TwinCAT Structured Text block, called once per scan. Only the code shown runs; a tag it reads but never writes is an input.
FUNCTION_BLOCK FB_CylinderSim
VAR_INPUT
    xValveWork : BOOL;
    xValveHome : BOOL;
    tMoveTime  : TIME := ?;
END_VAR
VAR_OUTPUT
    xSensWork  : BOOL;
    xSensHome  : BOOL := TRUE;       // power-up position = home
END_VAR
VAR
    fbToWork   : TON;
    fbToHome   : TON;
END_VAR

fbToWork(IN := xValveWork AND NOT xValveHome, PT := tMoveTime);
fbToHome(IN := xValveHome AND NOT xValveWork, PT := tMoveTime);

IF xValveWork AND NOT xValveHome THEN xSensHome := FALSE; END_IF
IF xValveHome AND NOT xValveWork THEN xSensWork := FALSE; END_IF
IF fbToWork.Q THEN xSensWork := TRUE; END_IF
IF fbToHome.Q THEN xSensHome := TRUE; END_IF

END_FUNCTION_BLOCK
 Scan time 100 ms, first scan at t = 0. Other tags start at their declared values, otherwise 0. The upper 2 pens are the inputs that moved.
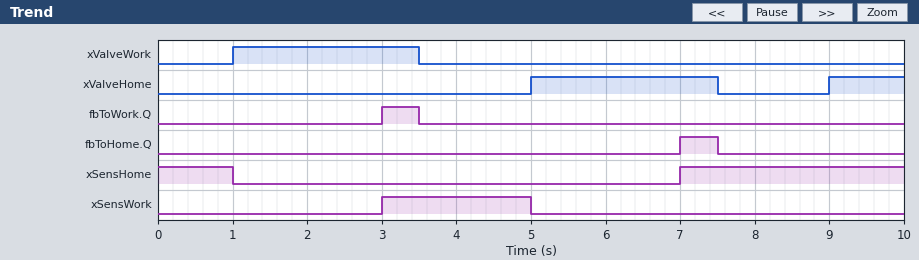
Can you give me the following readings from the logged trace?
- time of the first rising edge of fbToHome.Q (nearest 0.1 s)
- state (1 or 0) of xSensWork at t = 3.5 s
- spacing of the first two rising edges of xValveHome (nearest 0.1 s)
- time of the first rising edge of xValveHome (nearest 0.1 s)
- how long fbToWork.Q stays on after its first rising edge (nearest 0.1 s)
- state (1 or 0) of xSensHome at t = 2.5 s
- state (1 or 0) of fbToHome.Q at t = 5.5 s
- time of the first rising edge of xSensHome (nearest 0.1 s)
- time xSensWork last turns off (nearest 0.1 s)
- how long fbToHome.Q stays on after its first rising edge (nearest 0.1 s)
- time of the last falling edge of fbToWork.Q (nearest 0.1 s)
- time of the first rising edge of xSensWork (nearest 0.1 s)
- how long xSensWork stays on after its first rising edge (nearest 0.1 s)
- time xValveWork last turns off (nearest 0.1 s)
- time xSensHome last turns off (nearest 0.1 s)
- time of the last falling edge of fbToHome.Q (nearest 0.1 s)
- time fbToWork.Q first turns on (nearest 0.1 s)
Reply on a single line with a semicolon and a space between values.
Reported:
7.0 s; 1; 4.0 s; 5.0 s; 0.5 s; 0; 0; 7.0 s; 5.0 s; 0.5 s; 3.5 s; 3.0 s; 2.0 s; 3.5 s; 1.0 s; 7.5 s; 3.0 s
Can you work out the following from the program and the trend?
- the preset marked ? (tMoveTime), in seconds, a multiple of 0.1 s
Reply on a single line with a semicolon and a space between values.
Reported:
2.0 s
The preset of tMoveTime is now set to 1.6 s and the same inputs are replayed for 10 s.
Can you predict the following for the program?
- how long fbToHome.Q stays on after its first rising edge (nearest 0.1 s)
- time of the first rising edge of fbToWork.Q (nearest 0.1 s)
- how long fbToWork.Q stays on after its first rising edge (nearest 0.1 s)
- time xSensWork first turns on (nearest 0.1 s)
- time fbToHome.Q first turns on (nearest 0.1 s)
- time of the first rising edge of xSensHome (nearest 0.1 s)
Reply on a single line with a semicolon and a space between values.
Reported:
0.9 s; 2.6 s; 0.9 s; 2.6 s; 6.6 s; 6.6 s
